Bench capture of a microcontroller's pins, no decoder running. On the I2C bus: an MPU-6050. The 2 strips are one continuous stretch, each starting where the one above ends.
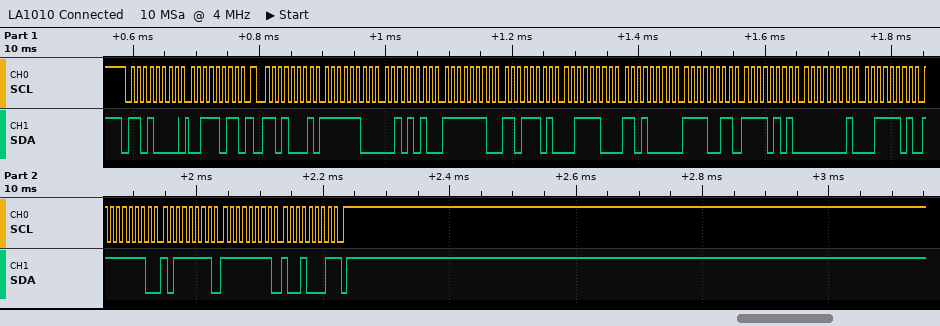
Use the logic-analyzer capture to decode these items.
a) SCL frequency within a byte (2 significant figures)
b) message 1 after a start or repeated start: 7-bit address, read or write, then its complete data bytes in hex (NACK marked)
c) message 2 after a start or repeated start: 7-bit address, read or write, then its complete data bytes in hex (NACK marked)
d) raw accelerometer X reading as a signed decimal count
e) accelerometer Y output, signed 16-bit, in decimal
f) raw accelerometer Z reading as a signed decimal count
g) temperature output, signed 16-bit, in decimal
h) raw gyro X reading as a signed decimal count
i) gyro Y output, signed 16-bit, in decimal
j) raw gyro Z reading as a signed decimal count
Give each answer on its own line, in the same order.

100 kHz
0x68 write: 3B
0x68 read: FC 2A FE DD 3C D0 F3 F5 01 3D FE BF FF 91 NACK
-982
-291
15568
-3083
317
-321
-111
